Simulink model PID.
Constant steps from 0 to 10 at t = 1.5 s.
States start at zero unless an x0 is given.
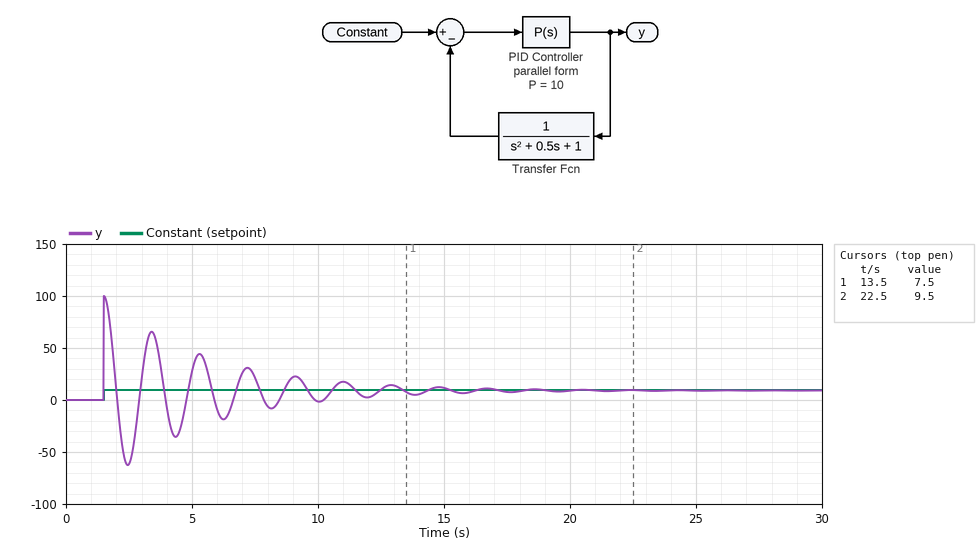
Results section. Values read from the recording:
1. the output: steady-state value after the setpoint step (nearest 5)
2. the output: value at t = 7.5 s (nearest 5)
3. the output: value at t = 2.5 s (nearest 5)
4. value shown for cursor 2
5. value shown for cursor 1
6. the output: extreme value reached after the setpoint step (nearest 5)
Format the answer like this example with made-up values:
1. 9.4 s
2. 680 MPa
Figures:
1. 10
2. 20
3. -60
4. 9.5
5. 7.5
6. 100
